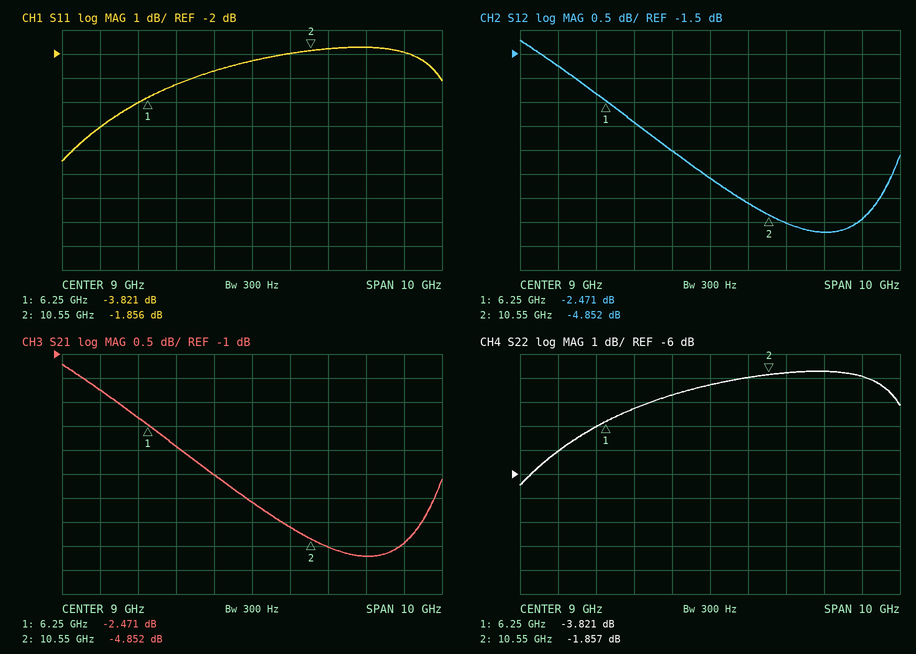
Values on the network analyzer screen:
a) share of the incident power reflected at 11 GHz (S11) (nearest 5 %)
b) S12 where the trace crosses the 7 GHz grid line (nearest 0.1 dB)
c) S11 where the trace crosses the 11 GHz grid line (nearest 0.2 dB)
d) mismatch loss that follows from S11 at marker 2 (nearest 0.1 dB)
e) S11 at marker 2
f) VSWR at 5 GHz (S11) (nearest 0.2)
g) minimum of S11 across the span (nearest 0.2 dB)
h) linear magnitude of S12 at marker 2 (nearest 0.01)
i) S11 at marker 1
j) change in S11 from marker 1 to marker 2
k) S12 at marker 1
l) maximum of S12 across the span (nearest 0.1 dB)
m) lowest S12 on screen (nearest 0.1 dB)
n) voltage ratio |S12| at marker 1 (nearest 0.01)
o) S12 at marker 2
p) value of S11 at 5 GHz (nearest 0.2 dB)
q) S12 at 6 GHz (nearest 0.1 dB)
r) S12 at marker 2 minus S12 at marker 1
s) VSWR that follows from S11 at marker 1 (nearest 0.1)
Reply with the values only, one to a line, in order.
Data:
65 %
-2.9 dB
-1.8 dB
4.6 dB
-1.856 dB
3.6
-6.4 dB
0.57
-3.821 dB
1.965 dB
-2.471 dB
-1.2 dB
-5.2 dB
0.75
-4.852 dB
-5.0 dB
-2.3 dB
-2.381 dB
4.6
